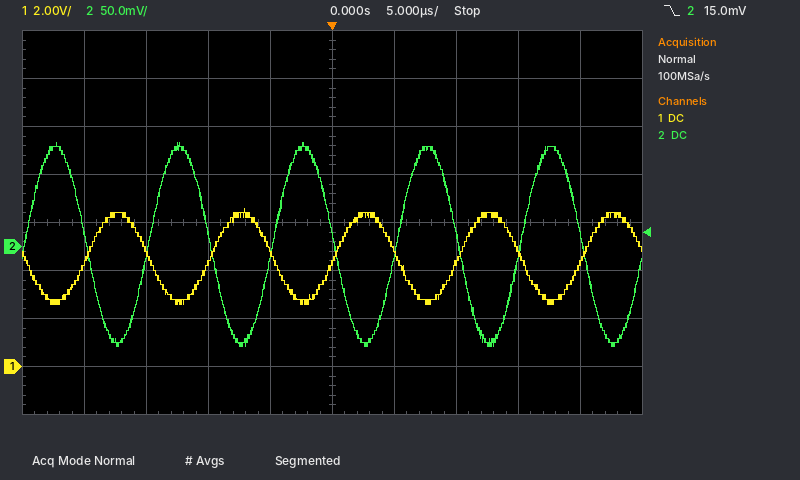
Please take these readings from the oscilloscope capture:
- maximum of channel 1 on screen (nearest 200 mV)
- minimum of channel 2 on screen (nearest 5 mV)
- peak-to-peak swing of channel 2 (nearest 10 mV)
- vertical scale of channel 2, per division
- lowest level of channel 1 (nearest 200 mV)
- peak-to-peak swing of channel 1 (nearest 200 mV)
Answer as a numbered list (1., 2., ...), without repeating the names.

1. 6.6 V
2. -105 mV
3. 210 mV
4. 50 mV
5. 2.6 V
6. 4.0 V
